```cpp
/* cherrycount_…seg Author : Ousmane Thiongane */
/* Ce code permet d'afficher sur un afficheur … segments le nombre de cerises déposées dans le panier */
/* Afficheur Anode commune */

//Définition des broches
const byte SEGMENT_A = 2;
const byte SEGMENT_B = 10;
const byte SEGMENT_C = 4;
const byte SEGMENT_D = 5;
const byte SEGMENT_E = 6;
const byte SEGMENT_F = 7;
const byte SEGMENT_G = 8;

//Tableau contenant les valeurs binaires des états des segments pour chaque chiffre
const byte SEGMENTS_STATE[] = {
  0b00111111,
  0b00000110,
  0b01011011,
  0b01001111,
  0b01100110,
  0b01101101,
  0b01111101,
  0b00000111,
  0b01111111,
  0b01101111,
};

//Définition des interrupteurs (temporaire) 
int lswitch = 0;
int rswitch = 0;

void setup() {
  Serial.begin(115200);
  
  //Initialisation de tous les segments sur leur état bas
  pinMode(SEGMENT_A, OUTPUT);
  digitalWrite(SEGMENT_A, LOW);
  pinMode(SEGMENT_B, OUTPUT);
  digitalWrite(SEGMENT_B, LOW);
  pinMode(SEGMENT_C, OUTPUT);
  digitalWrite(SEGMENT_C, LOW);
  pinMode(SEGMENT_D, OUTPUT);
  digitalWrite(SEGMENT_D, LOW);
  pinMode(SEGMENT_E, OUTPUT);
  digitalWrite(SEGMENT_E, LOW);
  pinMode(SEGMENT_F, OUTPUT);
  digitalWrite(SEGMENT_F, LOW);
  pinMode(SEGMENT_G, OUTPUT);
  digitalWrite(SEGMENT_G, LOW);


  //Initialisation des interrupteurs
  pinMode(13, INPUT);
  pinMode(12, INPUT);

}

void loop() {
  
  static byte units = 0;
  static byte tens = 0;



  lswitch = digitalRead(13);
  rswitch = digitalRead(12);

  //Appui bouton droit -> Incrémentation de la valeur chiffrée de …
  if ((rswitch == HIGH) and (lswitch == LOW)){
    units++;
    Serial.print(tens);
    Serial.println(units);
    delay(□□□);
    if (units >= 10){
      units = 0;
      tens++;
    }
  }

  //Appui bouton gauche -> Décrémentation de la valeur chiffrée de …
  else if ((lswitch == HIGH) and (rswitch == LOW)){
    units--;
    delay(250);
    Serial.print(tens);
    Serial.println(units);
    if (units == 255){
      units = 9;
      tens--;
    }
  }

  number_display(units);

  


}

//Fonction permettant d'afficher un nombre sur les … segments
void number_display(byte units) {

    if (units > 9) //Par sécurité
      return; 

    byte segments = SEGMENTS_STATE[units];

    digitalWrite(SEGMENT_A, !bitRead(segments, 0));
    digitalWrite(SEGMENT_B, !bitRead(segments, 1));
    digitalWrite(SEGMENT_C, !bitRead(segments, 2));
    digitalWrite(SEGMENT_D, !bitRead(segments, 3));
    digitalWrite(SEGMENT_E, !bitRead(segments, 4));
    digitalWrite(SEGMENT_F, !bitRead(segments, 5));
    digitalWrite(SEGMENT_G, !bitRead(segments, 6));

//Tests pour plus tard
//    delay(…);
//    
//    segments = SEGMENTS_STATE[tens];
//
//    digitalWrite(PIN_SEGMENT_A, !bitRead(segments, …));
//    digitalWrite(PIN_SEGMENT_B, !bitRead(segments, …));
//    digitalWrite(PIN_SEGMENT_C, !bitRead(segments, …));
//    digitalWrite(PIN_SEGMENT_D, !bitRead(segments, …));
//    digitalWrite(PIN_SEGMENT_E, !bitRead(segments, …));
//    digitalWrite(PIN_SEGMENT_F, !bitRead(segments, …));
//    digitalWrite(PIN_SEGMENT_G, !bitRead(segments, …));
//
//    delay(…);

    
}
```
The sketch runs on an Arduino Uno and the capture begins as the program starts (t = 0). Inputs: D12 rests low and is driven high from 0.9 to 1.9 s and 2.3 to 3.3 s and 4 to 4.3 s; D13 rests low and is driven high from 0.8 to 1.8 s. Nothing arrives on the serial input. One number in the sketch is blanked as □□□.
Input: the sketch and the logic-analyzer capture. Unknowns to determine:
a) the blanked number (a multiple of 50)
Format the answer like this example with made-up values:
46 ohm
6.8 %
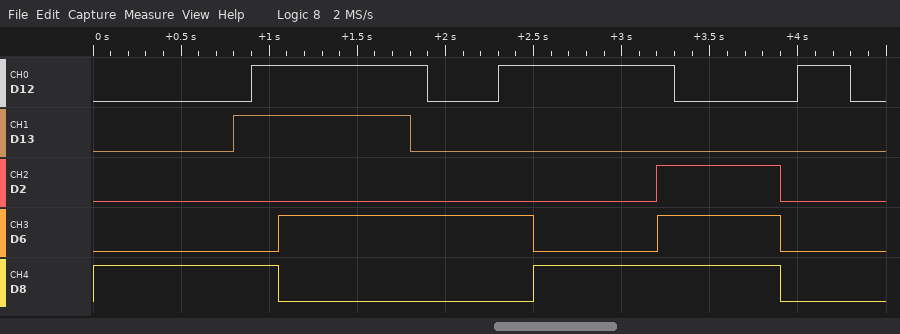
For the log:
700
